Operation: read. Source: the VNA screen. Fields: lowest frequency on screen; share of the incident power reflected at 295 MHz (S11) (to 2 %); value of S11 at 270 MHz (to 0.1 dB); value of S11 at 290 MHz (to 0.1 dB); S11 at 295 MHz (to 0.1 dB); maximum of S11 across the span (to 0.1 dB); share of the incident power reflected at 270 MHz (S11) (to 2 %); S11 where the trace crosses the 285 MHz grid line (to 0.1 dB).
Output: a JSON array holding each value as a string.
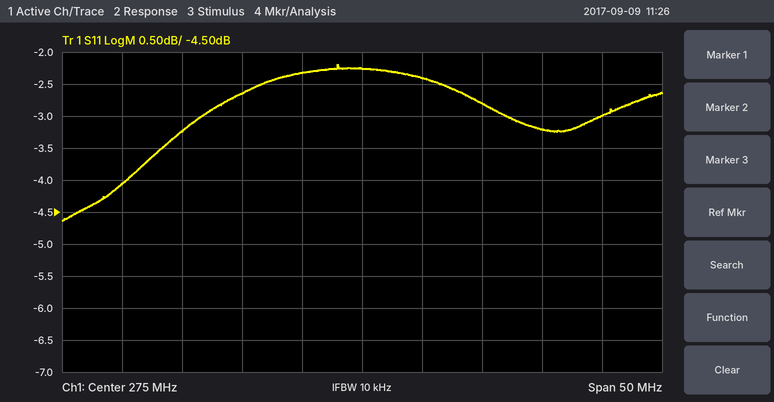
["250 MHz", "50 %", "-2.3 dB", "-3.2 dB", "-3.0 dB", "-2.2 dB", "58 %", "-2.8 dB"]
